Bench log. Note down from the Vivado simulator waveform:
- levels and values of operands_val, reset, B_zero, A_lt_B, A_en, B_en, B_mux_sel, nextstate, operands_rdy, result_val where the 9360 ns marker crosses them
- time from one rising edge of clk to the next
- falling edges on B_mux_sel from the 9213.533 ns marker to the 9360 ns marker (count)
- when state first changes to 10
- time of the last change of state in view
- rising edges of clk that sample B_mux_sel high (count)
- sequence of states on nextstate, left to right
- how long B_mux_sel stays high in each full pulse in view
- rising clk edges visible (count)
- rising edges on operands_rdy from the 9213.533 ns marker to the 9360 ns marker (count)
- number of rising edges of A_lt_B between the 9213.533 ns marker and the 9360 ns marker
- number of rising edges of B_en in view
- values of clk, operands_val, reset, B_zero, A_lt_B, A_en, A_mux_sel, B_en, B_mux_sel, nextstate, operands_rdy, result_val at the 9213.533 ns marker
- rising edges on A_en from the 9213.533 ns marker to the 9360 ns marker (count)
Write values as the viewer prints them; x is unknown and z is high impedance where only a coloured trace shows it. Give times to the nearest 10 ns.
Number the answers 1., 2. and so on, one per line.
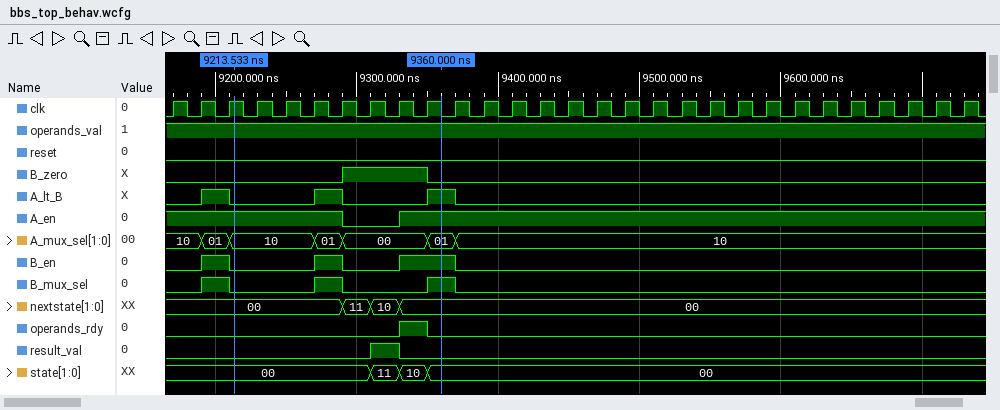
1. operands_val=1, reset=0, B_zero=0, A_lt_B=1, A_en=1, B_en=1, B_mux_sel=1, nextstate=00, operands_rdy=0, result_val=0
2. 20 ns
3. 1
4. 9330 ns
5. 9350 ns
6. 3
7. 00, 11, 10, 00
8. 20 ns, 20 ns, 20 ns
9. 29
10. 1
11. 2
12. 3
13. clk=1, operands_val=1, reset=0, B_zero=0, A_lt_B=0, A_en=1, A_mux_sel=10, B_en=0, B_mux_sel=0, nextstate=00, operands_rdy=0, result_val=0
14. 1
